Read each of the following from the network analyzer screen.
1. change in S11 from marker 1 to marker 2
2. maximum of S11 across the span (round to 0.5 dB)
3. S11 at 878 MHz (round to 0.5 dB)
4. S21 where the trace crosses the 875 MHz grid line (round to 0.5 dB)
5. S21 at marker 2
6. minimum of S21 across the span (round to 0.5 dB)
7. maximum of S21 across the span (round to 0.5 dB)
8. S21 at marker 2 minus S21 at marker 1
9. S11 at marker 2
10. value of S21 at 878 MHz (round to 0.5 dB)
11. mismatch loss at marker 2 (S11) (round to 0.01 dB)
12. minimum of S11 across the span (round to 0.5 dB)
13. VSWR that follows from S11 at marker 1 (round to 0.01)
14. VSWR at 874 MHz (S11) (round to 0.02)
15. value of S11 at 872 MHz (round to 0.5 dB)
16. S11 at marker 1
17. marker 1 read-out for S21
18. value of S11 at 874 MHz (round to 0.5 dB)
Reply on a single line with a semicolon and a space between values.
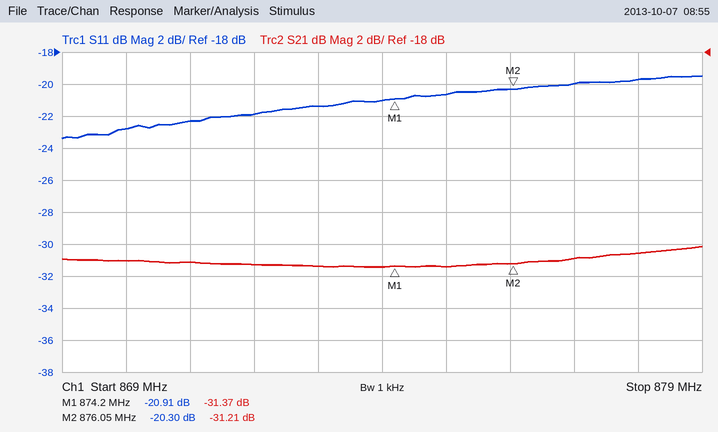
0.61 dB; -19.5 dB; -19.5 dB; -31.5 dB; -31.21 dB; -31.5 dB; -30.0 dB; 0.16 dB; -20.30 dB; -30.5 dB; 0.04 dB; -23.5 dB; 1.20; 1.20; -22.0 dB; -20.91 dB; -31.37 dB; -21.0 dB
